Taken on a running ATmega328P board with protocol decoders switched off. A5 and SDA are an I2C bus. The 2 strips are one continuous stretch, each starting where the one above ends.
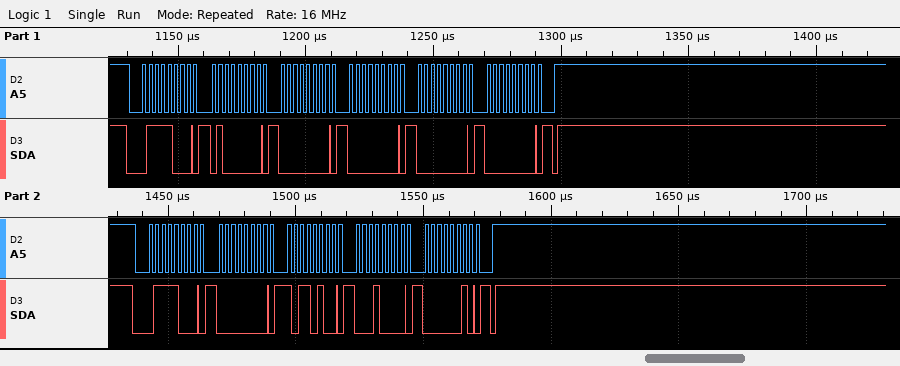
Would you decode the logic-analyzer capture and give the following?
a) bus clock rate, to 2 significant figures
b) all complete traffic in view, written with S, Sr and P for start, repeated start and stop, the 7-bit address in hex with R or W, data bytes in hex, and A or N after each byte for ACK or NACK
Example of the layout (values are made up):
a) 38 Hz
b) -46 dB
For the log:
a) 400 kHz
b) S 3CW A 40 A 00 A 00 A 00 A 00 A P S 3CW A 00 A B4 A 10 A 02 A P
